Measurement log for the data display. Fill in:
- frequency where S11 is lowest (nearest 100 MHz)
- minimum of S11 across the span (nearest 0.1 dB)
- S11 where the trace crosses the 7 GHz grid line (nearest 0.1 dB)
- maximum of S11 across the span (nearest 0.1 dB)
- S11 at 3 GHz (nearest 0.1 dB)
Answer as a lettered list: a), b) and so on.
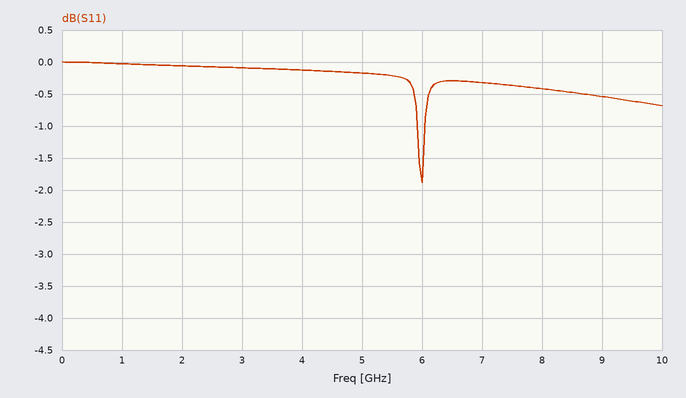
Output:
a) 6.0 GHz
b) -1.9 dB
c) -0.3 dB
d) 0.0 dB
e) -0.1 dB
